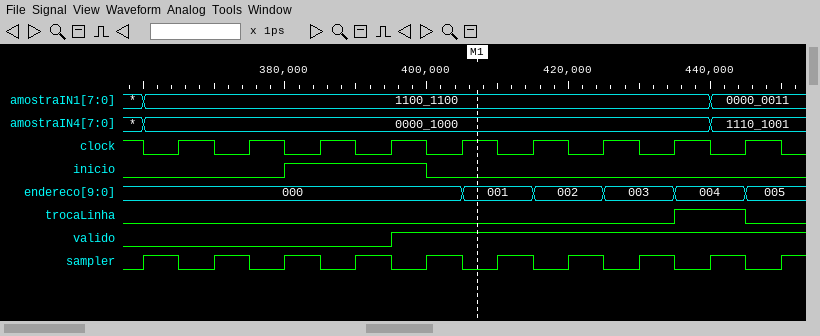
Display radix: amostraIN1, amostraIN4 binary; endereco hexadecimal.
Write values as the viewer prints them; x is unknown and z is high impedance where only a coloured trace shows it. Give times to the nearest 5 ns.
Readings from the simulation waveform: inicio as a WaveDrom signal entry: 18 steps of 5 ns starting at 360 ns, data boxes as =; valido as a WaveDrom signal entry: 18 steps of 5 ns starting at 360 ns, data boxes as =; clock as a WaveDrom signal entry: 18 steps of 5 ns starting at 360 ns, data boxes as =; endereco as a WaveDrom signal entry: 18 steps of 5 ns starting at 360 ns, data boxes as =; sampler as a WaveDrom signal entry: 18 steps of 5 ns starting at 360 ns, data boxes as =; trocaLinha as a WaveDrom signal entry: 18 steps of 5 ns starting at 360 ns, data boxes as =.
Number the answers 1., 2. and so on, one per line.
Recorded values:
1. {name: 'inicio', wave: '0...1...0.........'}
2. {name: 'valido', wave: '0......1..........'}
3. {name: 'clock', wave: '010101010101010101'}
4. {name: 'endereco', wave: '=........=.=.=.=.=', data: '000 001 002 003 004 005'}
5. {name: 'sampler', wave: '101010101010101010'}
6. {name: 'trocaLinha', wave: '0..............1.0'}
